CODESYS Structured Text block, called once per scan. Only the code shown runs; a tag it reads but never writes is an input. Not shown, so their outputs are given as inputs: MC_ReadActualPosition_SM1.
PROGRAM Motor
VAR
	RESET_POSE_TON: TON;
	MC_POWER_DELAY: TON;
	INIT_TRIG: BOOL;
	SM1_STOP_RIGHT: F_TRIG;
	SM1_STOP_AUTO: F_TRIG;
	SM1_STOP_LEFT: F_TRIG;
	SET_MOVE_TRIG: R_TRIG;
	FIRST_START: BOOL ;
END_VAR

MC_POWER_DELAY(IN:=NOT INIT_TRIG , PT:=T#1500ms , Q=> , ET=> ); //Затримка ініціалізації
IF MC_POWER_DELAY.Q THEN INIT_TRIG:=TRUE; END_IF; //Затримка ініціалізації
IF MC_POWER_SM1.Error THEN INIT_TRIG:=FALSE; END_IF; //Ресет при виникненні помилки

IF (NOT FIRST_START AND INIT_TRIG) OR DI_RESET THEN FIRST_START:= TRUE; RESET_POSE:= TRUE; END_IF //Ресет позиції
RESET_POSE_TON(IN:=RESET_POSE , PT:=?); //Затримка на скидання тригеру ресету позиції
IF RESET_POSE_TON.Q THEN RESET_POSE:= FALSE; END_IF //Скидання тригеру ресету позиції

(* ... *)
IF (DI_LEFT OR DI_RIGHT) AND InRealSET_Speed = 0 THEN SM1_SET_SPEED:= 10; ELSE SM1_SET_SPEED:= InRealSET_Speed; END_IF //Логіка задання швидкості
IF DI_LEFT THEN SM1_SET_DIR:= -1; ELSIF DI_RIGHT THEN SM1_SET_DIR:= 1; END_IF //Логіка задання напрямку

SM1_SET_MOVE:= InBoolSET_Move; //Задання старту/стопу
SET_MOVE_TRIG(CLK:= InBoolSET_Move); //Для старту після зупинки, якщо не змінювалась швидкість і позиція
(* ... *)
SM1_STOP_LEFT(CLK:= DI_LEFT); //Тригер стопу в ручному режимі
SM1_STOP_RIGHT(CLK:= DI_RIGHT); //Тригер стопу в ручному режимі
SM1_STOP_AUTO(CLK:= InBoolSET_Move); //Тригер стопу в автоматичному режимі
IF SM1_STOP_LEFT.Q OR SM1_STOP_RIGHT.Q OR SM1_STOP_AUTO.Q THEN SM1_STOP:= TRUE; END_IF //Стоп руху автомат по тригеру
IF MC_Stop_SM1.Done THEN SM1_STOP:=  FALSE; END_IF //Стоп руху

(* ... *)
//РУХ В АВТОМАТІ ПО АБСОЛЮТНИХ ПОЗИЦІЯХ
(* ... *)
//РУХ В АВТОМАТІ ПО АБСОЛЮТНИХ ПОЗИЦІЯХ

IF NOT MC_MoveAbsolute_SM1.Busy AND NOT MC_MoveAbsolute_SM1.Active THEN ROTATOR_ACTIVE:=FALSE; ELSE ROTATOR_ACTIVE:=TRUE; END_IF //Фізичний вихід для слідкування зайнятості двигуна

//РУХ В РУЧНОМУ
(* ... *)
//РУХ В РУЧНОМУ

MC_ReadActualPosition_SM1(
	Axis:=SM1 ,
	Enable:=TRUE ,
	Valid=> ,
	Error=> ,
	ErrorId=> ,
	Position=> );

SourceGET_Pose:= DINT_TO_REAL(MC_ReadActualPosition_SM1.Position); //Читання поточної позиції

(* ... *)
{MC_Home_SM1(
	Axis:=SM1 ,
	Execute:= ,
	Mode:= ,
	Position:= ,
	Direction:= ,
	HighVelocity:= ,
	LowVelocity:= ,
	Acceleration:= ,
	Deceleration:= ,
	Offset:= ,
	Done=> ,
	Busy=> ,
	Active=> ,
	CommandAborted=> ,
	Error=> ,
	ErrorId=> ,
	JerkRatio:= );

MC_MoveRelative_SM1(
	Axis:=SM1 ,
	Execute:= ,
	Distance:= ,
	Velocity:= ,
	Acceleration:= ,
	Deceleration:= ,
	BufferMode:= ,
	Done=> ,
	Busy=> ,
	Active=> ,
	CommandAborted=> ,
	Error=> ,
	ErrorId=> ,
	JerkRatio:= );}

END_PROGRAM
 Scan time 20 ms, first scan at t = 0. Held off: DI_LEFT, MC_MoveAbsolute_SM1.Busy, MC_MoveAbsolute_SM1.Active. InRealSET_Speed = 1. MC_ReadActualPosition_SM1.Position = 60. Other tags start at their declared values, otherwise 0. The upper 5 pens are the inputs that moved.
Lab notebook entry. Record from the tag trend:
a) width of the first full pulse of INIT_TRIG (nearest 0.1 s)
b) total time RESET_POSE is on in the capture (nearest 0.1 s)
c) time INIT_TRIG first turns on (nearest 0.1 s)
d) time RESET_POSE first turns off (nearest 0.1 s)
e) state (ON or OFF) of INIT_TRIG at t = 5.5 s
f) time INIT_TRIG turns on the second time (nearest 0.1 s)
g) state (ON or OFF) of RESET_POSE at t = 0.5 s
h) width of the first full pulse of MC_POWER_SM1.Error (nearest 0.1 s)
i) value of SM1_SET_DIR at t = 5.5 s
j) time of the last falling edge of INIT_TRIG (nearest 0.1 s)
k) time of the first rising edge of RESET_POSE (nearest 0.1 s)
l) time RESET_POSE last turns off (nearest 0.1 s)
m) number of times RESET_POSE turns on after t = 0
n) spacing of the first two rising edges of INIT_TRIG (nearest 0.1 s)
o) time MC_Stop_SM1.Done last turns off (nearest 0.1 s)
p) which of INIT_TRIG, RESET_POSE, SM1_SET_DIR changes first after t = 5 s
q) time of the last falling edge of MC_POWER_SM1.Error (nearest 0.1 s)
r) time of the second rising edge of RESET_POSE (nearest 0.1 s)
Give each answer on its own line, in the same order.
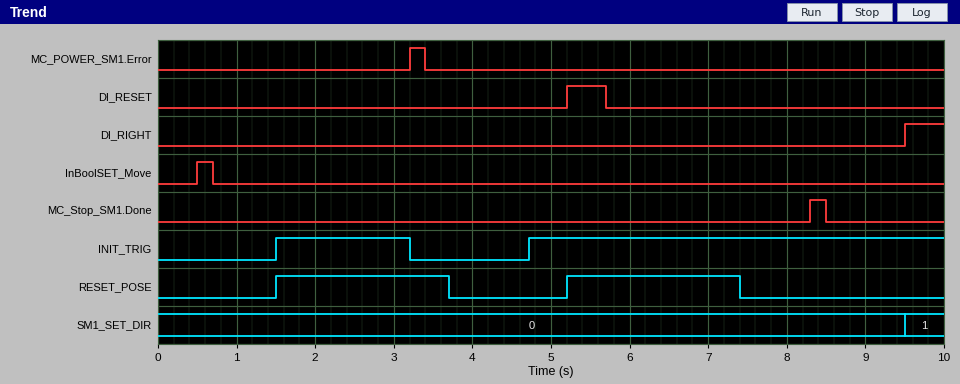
1.7 s
4.4 s
1.5 s
3.7 s
ON
4.7 s
OFF
0.2 s
0
3.2 s
1.5 s
7.4 s
2
3.2 s
8.5 s
RESET_POSE
3.4 s
5.2 s
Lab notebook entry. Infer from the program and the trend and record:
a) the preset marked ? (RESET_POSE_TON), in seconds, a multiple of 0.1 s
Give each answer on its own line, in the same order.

2.2 s
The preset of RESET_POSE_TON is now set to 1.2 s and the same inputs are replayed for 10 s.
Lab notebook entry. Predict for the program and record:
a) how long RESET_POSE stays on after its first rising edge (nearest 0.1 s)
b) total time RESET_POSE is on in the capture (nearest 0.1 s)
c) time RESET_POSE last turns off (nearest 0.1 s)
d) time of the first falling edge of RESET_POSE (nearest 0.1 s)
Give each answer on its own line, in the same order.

1.2 s
2.4 s
6.4 s
2.7 s
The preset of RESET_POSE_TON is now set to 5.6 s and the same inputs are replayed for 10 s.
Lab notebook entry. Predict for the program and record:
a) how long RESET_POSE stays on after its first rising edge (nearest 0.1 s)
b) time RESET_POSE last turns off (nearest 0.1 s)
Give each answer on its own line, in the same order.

5.6 s
7.1 s
